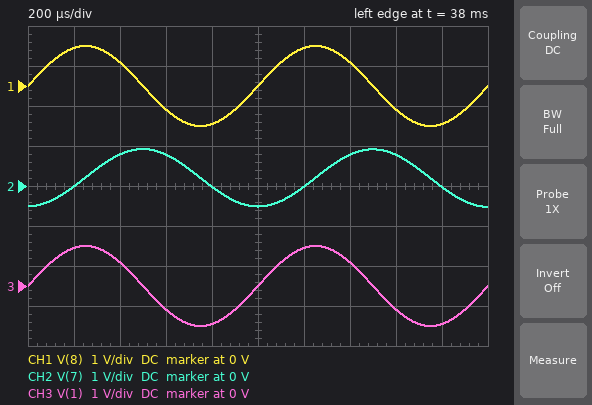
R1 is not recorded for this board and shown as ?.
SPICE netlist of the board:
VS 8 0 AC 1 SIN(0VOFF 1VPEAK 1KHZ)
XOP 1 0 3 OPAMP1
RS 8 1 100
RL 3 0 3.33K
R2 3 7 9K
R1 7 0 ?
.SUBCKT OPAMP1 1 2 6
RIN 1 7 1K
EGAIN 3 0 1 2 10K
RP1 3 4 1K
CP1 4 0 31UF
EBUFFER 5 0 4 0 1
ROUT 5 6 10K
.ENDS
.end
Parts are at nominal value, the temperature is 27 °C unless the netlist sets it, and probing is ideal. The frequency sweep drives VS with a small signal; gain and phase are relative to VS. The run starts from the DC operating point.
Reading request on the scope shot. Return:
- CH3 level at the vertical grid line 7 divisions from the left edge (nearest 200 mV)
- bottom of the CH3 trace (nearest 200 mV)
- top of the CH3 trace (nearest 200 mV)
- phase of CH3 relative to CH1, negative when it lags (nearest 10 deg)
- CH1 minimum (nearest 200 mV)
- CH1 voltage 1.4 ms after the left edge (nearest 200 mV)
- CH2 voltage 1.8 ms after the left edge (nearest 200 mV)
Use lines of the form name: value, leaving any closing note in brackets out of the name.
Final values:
CH3 level at the vertical grid line 7 divisions from the left edge: 600 mV
bottom of the CH3 trace: -1.0 V
top of the CH3 trace: 1.0 V
phase of CH3 relative to CH1, negative when it lags: 0 deg
CH1 minimum: -1.0 V
CH1 voltage 1.4 ms after the left edge: 600 mV
CH2 voltage 1.8 ms after the left edge: 0 V
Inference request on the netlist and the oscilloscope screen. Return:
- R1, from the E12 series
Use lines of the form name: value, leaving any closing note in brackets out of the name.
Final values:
R1, from the E12 series: 680 Ω
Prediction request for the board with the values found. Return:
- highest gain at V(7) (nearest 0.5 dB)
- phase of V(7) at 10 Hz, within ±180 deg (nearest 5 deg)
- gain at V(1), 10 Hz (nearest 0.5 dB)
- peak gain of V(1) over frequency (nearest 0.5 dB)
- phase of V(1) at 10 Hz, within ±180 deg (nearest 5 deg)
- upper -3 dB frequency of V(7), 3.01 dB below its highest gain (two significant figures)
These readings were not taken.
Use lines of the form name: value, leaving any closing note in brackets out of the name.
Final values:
highest gain at V(7): 43.0 dB
phase of V(7) at 10 Hz, within ±180 deg: -65 deg
gain at V(1), 10 Hz: 0 dB
peak gain of V(1) over frequency: 0 dB
phase of V(1) at 10 Hz, within ±180 deg: 0 deg
upper -3 dB frequency of V(7), 3.01 dB below its highest gain: 5.1 Hz
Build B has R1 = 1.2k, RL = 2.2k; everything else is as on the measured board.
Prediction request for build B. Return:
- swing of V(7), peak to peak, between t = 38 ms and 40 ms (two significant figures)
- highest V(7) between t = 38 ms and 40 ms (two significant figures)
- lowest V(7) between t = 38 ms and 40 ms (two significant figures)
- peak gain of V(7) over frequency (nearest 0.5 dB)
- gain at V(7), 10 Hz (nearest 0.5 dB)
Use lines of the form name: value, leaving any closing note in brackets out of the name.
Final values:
swing of V(7), peak to peak, between t = 38 ms and 40 ms: 1.9 V
highest V(7) between t = 38 ms and 40 ms: 1.2 V
lowest V(7) between t = 38 ms and 40 ms: -670 mV
peak gain of V(7) over frequency: 45.0 dB
gain at V(7), 10 Hz: 38.5 dB
